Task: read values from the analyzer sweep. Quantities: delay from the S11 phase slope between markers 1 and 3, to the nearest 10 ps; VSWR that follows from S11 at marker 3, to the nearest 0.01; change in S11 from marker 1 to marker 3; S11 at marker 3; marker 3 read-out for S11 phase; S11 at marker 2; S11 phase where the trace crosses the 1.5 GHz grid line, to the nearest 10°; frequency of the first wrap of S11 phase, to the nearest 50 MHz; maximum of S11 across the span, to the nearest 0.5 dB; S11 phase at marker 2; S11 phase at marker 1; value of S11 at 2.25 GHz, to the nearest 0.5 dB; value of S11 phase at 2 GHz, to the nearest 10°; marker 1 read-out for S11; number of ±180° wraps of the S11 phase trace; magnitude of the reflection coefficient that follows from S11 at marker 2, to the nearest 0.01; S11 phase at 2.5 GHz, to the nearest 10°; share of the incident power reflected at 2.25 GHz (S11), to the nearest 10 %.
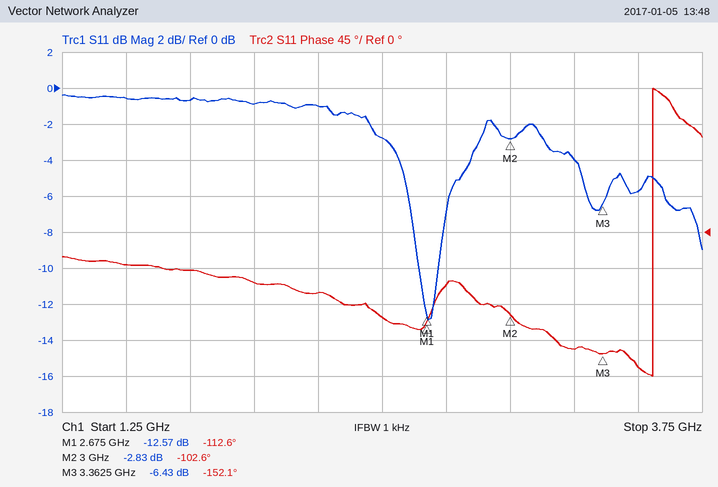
160 ps
2.82
6.14 dB
-6.43 dB
-152.1°
-2.83 dB
-40°
3.55 GHz
-0.5 dB
-102.6°
-112.6°
-1.0 dB
-60°
-12.57 dB
1
0.72
-110°
80 %
